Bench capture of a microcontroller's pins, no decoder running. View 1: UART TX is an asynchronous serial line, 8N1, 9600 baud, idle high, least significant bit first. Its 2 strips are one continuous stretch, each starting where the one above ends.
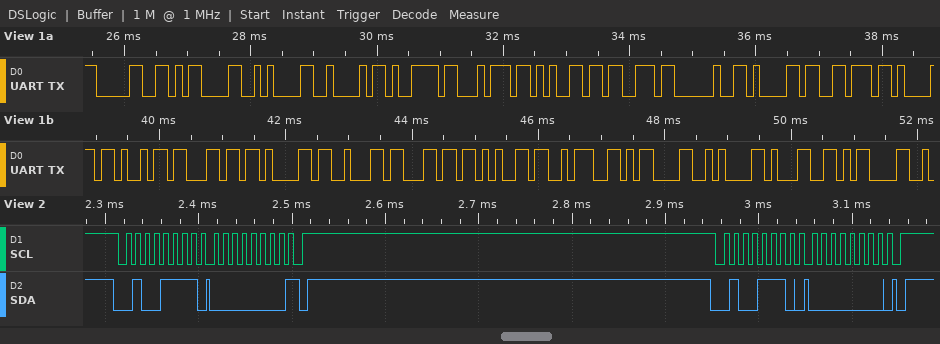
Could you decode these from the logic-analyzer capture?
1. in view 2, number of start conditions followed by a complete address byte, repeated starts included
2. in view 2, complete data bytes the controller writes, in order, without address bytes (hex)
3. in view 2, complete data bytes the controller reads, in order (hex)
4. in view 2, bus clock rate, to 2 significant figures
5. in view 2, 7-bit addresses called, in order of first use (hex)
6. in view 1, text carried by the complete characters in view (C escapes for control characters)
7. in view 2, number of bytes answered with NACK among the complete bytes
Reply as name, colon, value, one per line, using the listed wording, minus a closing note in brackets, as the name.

in view 2, number of start conditions followed by a complete address byte, repeated starts included: 2
in view 2, complete data bytes the controller writes, in order, without address bytes: 00
in view 2, complete data bytes the controller reads, in order: 00
in view 2, bus clock rate, to 2 significant figures: 100 kHz
in view 2, 7-bit addresses called, in order of first use: 0x27
in view 1, text carried by the complete characters in view: "0\r\nBytes available:\r\n1\r"
in view 2, number of bytes answered with NACK among the complete bytes: 1
